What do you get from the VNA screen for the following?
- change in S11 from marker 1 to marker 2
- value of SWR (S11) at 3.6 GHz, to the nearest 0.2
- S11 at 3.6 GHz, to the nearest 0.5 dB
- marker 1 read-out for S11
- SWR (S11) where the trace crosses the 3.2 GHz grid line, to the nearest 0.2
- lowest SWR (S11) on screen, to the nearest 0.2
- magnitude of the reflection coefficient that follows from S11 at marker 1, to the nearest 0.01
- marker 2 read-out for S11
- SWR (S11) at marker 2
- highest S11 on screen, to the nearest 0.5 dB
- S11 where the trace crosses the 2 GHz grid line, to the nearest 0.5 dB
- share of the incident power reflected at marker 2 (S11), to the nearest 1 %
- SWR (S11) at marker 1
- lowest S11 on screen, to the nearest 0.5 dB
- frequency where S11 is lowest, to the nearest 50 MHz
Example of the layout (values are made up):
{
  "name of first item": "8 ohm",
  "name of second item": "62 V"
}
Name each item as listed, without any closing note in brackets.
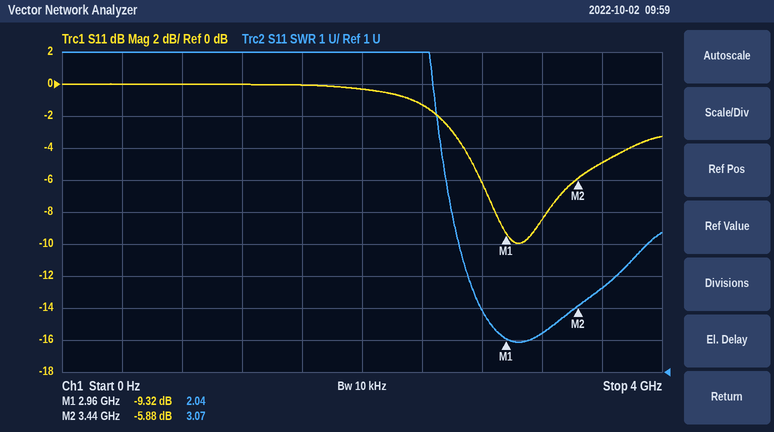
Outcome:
{
  "change in S11 from marker 1 to marker 2": "3.44 dB",
  "value of SWR (S11) at 3.6 GHz, to the nearest 0.2": "3.6",
  "S11 at 3.6 GHz, to the nearest 0.5 dB": "-5.0 dB",
  "marker 1 read-out for S11": "-9.32 dB",
  "SWR (S11) where the trace crosses the 3.2 GHz grid line, to the nearest 0.2": "2.2",
  "lowest SWR (S11) on screen, to the nearest 0.2": "2.0",
  "magnitude of the reflection coefficient that follows from S11 at marker 1, to the nearest 0.01": "0.34",
  "marker 2 read-out for S11": "-5.88 dB",
  "SWR (S11) at marker 2": "3.07",
  "highest S11 on screen, to the nearest 0.5 dB": "0.0 dB",
  "S11 where the trace crosses the 2 GHz grid line, to the nearest 0.5 dB": "-0.5 dB",
  "share of the incident power reflected at marker 2 (S11), to the nearest 1 %": "26 %",
  "SWR (S11) at marker 1": "2.04",
  "lowest S11 on screen, to the nearest 0.5 dB": "-10.0 dB",
  "frequency where S11 is lowest, to the nearest 50 MHz": "3.05 GHz"
}
